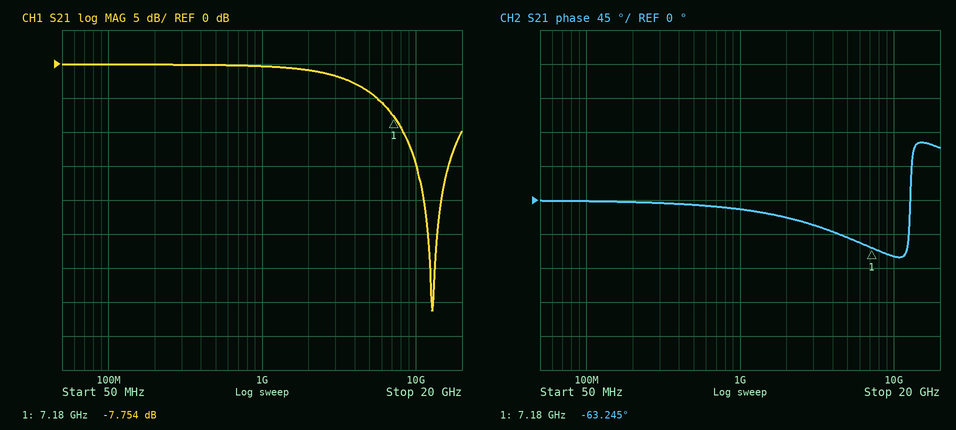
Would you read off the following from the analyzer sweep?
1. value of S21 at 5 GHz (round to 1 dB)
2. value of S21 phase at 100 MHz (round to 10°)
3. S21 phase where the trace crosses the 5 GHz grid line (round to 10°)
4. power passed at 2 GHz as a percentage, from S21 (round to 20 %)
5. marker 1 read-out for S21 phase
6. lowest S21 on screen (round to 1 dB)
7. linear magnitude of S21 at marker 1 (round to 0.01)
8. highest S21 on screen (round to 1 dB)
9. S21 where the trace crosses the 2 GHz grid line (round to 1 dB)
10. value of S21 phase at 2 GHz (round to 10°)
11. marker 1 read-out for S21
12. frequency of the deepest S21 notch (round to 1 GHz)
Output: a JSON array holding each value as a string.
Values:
["-4 dB", "0°", "-50°", "80 %", "-63.245°", "-36 dB", "0.41", "0 dB", "-1 dB", "-20°", "-7.754 dB", "13 GHz"]
